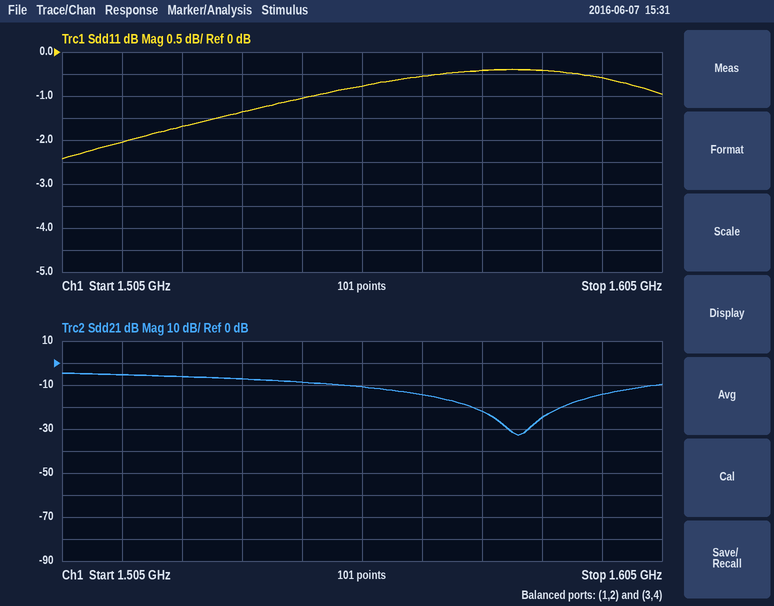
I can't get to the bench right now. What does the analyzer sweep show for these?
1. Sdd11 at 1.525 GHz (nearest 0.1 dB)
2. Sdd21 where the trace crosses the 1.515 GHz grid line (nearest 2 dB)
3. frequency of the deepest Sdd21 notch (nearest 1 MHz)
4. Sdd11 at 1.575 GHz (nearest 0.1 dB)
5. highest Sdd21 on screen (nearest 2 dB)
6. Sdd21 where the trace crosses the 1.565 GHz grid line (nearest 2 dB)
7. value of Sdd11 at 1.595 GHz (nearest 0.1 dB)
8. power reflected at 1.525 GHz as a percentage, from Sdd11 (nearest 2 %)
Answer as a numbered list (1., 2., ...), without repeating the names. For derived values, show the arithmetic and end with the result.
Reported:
1. -1.7 dB
2. -6 dB
3. 1.581 GHz
4. -0.4 dB
5. -4 dB
6. -14 dB
7. -0.6 dB
8. 10^(-1.7/10) ≈ 68 %
